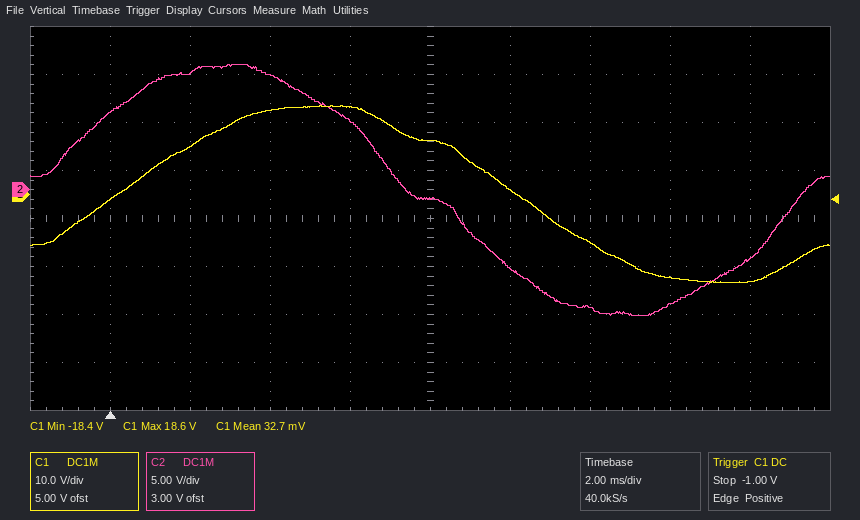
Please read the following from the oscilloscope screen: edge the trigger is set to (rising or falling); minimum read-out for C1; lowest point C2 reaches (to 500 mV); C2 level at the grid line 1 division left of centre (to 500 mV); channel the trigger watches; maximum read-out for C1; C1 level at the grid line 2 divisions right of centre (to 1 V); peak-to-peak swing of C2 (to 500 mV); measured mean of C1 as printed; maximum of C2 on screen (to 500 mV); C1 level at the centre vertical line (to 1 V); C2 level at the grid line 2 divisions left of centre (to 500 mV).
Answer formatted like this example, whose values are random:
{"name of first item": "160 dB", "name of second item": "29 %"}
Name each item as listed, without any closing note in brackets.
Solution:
{"edge the trigger is set to": "rising", "minimum read-out for C1": "-18.4 V", "lowest point C2 reaches": "-13.0 V", "C2 level at the grid line 1 division left of centre": "7.0 V", "channel the trigger watches": "C1", "maximum read-out for C1": "18.6 V", "C1 level at the grid line 2 divisions right of centre": "-10 V", "peak-to-peak swing of C2": "26.0 V", "measured mean of C1 as printed": "32.7 mV", "maximum of C2 on screen": "13.0 V", "C1 level at the centre vertical line": "11 V", "C2 level at the grid line 2 divisions left of centre": "12.0 V"}
